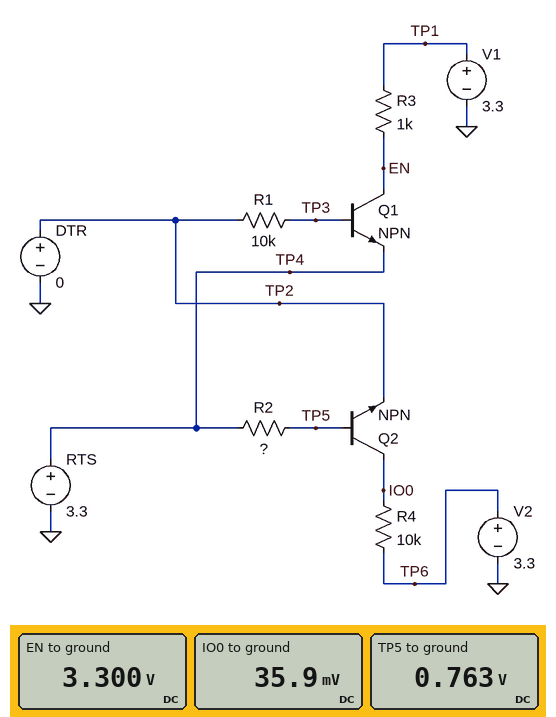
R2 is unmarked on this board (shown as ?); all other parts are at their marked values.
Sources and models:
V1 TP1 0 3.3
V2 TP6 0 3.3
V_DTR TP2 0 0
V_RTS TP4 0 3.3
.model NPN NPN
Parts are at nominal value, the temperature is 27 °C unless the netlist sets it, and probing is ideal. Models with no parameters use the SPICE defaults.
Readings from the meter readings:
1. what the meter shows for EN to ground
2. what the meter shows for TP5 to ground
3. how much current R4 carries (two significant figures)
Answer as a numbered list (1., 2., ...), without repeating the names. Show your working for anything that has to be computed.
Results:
1. 3.300 V
2. 0.763 V
3. (3.3 V - 35.9 mV) / 10 kΩ = 330 µA
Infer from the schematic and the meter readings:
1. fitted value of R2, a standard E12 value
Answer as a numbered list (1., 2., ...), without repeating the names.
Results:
1. 15 kΩ
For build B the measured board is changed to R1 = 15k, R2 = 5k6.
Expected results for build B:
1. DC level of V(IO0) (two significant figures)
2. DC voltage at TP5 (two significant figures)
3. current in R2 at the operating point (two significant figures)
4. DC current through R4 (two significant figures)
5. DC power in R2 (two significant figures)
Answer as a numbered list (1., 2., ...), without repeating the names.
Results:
1. 26 mV
2. 780 mV
3. 450 µA
4. 330 µA
5. 1.1 mW
